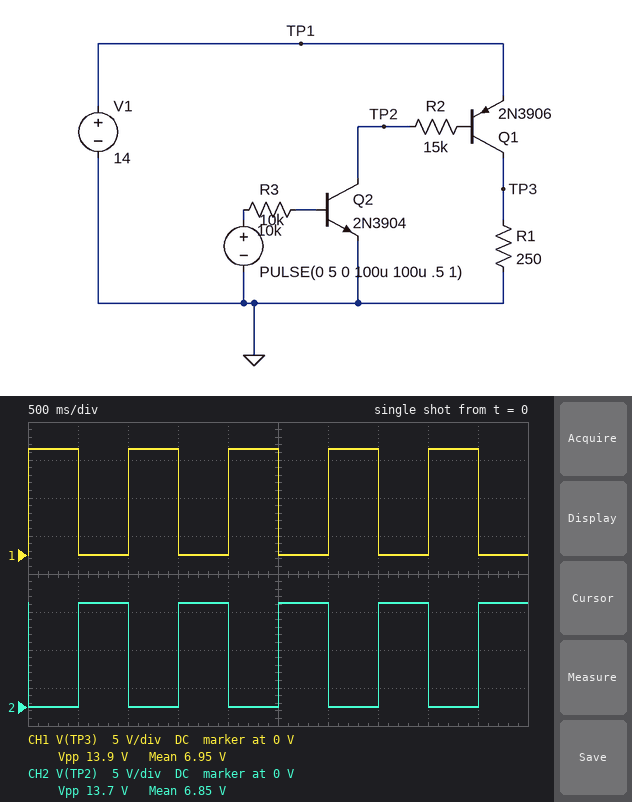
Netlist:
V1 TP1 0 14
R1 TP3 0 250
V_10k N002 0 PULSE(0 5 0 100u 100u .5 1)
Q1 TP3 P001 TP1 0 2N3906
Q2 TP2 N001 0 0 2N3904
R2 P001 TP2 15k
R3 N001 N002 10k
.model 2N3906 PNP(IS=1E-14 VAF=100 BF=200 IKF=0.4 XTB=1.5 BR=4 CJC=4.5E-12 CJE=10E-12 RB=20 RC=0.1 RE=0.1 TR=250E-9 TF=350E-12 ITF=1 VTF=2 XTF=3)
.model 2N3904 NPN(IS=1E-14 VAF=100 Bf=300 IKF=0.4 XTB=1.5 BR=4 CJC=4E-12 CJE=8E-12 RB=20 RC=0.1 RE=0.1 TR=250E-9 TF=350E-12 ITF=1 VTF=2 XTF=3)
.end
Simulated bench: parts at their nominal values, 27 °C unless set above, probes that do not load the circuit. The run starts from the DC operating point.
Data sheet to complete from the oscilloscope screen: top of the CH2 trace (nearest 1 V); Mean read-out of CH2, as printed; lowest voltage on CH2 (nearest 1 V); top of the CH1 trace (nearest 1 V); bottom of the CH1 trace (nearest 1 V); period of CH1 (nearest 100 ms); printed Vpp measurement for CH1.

14 V
6.85 V
0 V
14 V
0 V
1.0 s
13.9 V
